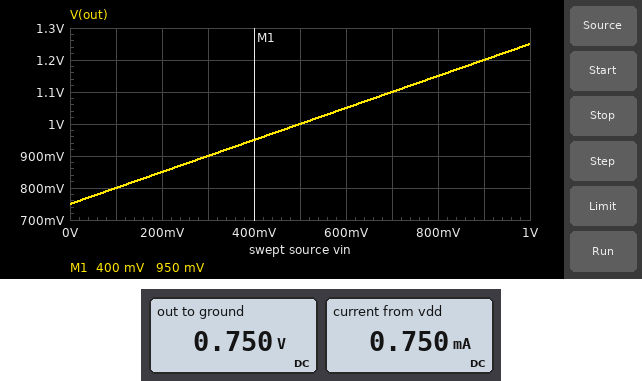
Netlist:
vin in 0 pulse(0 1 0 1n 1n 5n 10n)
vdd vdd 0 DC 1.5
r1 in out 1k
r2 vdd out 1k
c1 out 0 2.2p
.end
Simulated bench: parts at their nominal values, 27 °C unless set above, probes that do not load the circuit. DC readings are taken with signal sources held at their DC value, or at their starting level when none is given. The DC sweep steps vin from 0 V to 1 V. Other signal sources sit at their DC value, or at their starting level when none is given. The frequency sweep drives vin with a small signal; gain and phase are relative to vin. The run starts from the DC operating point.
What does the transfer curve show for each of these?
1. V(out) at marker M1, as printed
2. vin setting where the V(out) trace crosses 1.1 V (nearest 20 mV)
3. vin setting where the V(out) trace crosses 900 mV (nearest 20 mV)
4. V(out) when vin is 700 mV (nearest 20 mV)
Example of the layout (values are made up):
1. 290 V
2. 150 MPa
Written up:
1. 950 mV
2. 700 mV
3. 300 mV
4. 1.10 V
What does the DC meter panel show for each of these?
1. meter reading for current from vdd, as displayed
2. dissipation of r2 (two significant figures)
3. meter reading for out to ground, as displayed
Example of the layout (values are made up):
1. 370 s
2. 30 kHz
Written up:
1. 0.750 mA
2. 560 µW
3. 0.750 V
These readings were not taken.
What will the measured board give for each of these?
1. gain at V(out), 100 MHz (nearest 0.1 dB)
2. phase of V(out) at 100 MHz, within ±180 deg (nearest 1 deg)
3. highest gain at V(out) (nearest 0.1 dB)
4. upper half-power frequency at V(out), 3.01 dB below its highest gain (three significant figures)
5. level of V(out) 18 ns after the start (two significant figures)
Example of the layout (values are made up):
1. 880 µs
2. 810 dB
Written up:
1. -7.7 dB
2. -35 deg
3. -6.0 dB
4. 145 MHz
5. 880 mV
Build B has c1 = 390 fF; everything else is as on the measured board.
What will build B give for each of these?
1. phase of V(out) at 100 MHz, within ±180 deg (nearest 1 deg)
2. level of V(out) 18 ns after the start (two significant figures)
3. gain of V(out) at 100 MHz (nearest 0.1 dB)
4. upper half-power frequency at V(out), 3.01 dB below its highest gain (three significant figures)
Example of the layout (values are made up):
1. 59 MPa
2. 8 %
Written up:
1. -7 deg
2. 750 mV
3. -6.1 dB
4. 816 MHz
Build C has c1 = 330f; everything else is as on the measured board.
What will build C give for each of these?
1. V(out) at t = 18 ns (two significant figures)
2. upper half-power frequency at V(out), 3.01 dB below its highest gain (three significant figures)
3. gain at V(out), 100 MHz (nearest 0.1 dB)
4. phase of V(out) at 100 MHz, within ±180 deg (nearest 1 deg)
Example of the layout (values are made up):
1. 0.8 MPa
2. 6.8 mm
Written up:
1. 750 mV
2. 965 MHz
3. -6.1 dB
4. -6 deg
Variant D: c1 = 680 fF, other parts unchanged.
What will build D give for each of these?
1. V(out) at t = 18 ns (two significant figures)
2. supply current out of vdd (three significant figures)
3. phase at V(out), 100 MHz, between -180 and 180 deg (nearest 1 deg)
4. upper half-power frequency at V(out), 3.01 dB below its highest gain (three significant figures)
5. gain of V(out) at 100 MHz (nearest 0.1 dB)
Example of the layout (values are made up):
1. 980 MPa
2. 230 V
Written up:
1. 760 mV
2. 750 µA
3. -12 deg
4. 468 MHz
5. -6.2 dB
